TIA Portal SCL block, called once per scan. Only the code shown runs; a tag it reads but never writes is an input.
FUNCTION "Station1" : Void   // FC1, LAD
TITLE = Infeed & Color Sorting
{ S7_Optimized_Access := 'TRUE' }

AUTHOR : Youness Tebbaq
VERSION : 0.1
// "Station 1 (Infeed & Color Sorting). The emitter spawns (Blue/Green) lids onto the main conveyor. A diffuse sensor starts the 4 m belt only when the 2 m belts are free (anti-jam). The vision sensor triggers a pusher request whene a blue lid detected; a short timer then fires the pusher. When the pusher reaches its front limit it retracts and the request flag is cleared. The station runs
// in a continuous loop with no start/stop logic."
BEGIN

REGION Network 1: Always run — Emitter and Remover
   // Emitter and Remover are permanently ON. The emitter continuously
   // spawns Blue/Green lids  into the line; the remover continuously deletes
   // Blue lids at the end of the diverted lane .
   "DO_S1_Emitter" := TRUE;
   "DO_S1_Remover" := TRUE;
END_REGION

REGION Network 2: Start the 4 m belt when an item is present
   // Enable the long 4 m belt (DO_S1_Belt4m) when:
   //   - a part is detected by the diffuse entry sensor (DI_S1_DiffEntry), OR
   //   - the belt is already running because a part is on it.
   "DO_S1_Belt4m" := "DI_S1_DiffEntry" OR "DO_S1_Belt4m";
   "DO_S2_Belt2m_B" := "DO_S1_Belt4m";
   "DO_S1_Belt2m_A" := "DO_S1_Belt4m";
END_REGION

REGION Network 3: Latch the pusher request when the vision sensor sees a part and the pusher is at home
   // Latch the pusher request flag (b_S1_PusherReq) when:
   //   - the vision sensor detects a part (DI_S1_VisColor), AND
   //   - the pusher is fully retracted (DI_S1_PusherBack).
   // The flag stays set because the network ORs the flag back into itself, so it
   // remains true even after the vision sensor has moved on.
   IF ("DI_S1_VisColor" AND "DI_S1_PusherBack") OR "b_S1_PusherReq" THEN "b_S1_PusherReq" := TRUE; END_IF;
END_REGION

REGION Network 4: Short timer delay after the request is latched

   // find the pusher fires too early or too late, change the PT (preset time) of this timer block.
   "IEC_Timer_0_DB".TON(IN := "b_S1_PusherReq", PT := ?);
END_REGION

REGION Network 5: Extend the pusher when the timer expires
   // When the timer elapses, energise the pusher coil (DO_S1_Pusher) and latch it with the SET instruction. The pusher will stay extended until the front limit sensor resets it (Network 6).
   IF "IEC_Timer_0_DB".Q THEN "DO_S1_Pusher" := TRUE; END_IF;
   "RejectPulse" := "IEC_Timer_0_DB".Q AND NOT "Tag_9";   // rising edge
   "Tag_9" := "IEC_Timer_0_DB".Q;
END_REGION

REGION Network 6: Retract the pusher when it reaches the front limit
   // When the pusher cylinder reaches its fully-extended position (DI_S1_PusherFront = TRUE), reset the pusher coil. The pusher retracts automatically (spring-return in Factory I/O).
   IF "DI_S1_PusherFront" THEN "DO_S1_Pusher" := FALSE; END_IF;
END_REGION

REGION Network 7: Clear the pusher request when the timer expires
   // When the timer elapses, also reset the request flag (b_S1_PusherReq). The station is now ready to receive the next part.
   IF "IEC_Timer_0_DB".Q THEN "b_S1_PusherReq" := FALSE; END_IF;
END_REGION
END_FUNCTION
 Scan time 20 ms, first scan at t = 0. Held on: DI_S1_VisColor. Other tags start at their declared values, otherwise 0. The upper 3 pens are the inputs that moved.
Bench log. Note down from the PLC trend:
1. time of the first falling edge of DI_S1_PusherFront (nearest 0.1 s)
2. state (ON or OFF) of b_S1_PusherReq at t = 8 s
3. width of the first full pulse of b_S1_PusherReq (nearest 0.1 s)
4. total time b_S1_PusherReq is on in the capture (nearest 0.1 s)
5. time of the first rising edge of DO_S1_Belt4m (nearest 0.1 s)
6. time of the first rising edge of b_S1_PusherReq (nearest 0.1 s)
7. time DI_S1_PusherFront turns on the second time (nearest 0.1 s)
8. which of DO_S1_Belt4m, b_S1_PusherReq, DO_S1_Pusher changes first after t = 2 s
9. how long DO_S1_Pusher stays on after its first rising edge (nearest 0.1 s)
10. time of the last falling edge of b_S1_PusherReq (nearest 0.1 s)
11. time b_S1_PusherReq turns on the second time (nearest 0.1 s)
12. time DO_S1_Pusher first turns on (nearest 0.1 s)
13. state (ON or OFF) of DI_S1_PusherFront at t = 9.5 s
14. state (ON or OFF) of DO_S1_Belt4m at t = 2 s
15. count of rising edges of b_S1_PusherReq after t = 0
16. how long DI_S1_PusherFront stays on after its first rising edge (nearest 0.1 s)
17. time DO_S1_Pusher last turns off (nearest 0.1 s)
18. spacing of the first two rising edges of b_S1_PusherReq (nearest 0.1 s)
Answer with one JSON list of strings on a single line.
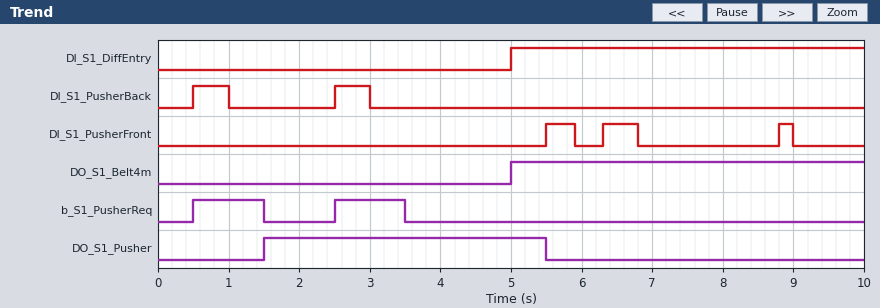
["5.9 s", "OFF", "1.0 s", "2.0 s", "5.0 s", "0.5 s", "6.3 s", "b_S1_PusherReq", "4.0 s", "3.5 s", "2.5 s", "1.5 s", "OFF", "OFF", "2", "0.4 s", "5.5 s", "2.0 s"]
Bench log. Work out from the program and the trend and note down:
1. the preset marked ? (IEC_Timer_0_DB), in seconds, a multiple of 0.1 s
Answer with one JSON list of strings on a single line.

["1.0 s"]
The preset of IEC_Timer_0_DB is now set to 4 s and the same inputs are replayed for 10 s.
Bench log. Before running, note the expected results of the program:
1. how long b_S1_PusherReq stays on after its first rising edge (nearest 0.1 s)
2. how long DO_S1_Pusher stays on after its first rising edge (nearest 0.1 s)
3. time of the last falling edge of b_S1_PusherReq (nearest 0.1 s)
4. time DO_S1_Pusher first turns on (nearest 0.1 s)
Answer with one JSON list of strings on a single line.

["4.0 s", "1.0 s", "4.5 s", "4.5 s"]
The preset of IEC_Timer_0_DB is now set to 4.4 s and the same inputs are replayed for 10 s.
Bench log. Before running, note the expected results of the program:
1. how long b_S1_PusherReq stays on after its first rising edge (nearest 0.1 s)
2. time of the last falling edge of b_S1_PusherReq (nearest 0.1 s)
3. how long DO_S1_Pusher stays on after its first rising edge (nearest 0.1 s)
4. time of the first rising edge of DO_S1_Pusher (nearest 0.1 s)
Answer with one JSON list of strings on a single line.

["4.4 s", "4.9 s", "0.6 s", "4.9 s"]
